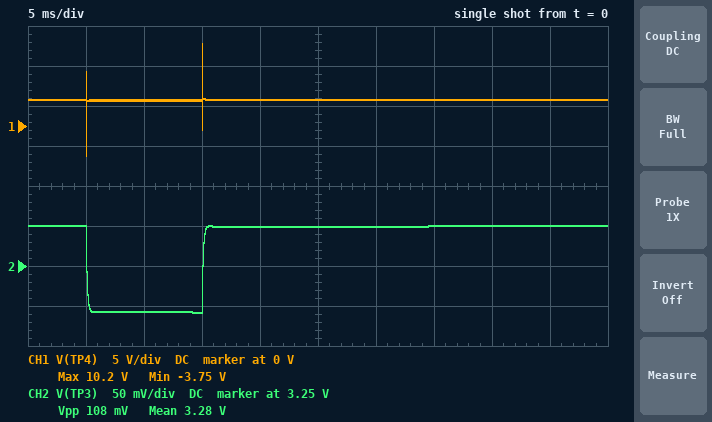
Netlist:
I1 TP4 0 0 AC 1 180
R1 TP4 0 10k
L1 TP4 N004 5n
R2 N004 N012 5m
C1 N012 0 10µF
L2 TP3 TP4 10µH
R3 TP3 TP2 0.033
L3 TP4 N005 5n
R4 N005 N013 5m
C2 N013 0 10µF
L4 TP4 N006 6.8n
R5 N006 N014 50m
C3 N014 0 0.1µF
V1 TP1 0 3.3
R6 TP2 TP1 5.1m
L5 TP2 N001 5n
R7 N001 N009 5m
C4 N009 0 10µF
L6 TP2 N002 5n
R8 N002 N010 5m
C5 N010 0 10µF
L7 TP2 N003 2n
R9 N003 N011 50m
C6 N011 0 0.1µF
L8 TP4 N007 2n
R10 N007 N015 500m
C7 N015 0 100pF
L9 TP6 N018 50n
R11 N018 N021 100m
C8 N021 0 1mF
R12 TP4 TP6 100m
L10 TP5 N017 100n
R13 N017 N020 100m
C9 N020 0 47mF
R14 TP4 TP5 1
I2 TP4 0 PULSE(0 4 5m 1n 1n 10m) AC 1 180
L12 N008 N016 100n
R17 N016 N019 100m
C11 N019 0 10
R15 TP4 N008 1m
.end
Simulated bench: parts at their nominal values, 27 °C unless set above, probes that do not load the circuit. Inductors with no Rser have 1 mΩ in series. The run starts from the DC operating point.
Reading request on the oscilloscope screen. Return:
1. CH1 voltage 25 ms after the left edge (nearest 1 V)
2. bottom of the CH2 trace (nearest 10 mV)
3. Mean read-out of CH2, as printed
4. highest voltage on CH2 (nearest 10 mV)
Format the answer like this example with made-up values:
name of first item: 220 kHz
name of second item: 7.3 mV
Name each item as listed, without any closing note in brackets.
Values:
CH1 voltage 25 ms after the left edge: 3 V
bottom of the CH2 trace: 3.19 V
Mean read-out of CH2, as printed: 3.28 V
highest voltage on CH2: 3.30 V
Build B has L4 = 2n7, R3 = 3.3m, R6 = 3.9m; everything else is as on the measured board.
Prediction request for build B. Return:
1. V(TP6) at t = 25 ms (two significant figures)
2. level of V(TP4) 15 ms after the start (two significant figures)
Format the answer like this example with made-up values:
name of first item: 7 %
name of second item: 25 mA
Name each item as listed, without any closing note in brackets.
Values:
V(TP6) at t = 25 ms: 3.3 V
level of V(TP4) 15 ms after the start: 3.3 V
